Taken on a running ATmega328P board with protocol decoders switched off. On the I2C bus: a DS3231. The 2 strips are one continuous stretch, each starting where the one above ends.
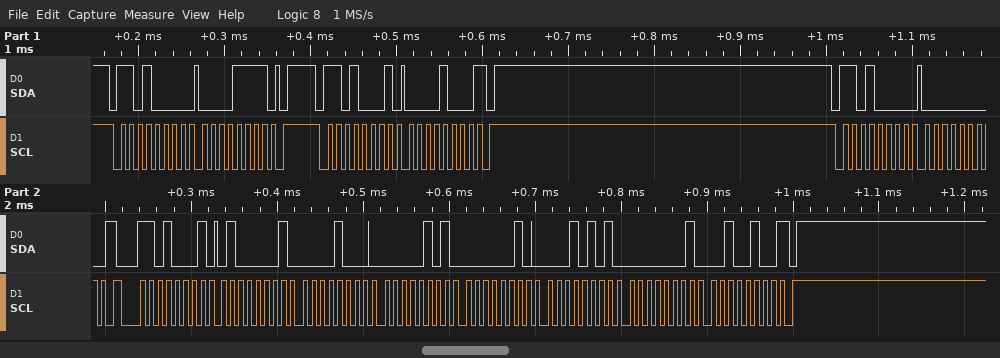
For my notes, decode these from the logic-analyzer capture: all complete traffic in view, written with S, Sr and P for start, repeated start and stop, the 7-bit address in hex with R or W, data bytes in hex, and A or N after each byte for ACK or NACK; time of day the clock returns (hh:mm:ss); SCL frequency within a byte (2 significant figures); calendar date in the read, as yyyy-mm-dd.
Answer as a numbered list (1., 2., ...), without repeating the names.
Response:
1. S 68W A 0F A P S 68R A 08 N P S 68W A 00 A Sr 68R A 41 A 08 A 05 A 02 A 15 A 01 A 24 N P
2. 05:08:41
3. 100 kHz
4. 2024-01-15
